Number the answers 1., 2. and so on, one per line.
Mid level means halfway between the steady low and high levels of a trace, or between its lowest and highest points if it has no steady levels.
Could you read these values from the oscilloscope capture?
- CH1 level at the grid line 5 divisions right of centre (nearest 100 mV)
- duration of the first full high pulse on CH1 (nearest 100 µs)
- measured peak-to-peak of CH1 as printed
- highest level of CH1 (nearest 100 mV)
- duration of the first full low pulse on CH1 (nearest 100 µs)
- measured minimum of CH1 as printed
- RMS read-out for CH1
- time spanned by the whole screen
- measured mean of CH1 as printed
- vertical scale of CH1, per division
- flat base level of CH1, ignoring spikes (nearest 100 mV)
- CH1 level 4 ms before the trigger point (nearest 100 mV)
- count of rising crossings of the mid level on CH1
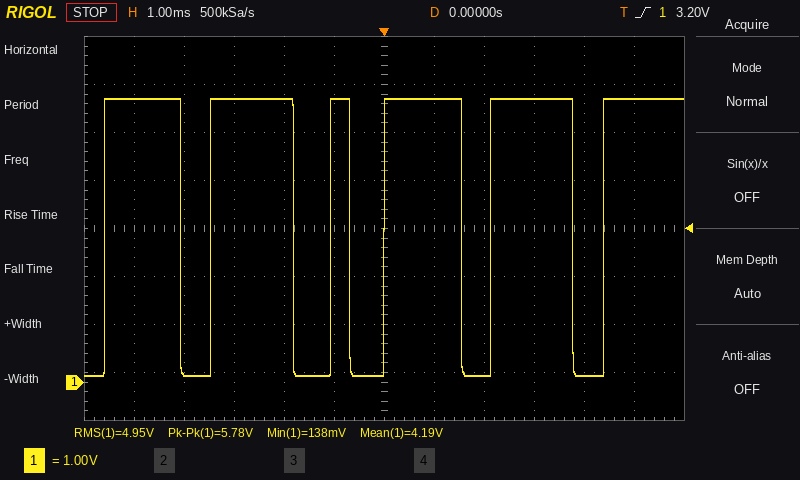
1. 5.9 V
2. 1.5 ms
3. 5.78 V
4. 5.9 V
5. 600 µs
6. 138 mV
7. 4.95 V
8. 12 ms
9. 4.19 V
10. 1 V
11. 100 mV
12. 200 mV
13. 6
